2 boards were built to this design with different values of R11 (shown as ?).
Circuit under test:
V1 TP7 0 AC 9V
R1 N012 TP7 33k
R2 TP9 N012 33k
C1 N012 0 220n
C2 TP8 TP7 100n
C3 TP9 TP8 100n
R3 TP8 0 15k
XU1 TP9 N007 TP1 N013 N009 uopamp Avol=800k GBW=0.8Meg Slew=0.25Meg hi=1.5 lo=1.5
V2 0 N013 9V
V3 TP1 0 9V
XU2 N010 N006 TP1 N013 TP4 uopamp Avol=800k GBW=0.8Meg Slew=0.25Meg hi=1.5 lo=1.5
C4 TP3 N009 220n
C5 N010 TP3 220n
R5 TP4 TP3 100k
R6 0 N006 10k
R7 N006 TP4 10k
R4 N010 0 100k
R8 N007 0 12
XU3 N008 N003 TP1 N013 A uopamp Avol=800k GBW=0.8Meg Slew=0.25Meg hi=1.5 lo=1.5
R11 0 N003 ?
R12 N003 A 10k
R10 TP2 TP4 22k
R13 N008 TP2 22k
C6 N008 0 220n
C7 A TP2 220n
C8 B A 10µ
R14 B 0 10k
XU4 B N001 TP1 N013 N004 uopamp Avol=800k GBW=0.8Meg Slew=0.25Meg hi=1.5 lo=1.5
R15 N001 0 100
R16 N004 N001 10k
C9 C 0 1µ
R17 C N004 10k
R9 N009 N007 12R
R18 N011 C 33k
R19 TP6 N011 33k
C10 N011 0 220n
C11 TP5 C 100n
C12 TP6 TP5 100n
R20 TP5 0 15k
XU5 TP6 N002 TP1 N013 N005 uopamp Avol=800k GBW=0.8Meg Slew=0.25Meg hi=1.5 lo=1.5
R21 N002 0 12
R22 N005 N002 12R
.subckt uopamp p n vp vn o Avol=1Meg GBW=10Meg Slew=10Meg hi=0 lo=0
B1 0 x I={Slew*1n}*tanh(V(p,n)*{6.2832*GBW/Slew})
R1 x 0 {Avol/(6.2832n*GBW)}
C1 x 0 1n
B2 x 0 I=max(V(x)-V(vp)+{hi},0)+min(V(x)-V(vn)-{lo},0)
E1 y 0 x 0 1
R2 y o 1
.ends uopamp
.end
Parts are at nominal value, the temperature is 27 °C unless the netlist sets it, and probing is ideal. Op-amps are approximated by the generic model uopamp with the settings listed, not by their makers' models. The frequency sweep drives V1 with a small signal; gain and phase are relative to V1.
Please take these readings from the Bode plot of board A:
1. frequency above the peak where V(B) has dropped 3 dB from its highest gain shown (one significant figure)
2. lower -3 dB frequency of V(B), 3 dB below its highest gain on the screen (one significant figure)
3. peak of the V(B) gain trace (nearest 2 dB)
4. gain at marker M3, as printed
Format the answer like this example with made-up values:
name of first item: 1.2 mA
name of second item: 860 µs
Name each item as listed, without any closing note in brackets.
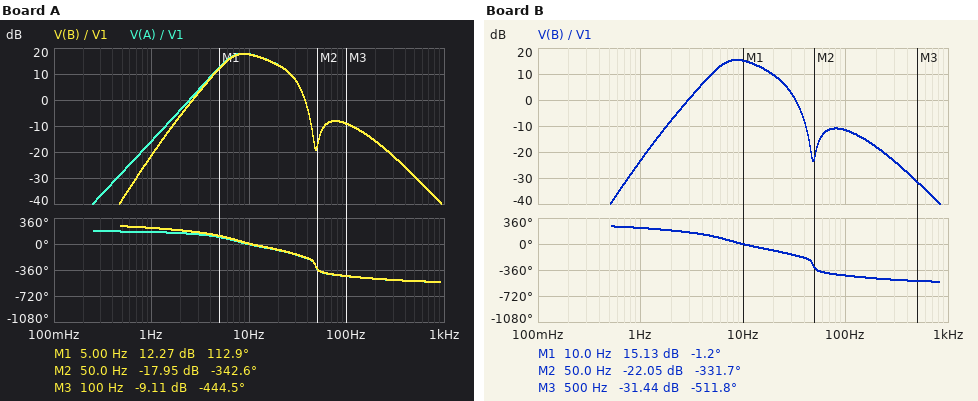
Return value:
frequency above the peak where V(B) has dropped 3 dB from its highest gain shown: 20 Hz
lower -3 dB frequency of V(B), 3 dB below its highest gain on the screen: 6 Hz
peak of the V(B) gain trace: 18 dB
gain at marker M3, as printed: -9.11 dB
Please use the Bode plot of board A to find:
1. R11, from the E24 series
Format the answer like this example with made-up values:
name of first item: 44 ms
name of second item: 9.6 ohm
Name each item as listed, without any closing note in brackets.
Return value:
R11, from the E24 series: 9.1 kΩ
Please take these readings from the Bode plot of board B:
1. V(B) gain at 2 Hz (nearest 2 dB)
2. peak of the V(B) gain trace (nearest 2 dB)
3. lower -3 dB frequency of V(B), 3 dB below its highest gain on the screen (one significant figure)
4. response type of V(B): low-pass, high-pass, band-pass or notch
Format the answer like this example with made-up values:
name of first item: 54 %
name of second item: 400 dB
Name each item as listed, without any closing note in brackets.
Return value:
V(B) gain at 2 Hz: -8 dB
peak of the V(B) gain trace: 16 dB
lower -3 dB frequency of V(B), 3 dB below its highest gain on the screen: 6 Hz
response type of V(B): low-pass, high-pass, band-pass or notch: band-pass
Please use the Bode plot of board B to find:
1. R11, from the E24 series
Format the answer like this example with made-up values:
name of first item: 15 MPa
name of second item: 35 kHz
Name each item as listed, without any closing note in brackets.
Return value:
R11, from the E24 series: 15 kΩ
